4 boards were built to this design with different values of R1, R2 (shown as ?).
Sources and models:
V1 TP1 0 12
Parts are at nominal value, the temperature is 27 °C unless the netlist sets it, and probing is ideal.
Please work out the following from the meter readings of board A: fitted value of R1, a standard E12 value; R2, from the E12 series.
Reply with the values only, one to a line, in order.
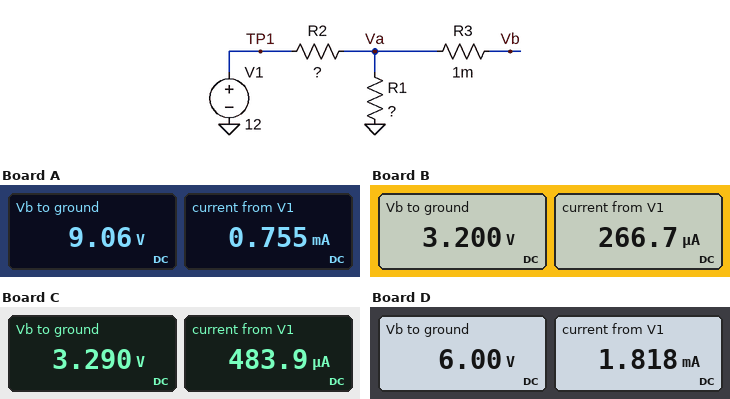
12 kΩ
3.9 kΩ
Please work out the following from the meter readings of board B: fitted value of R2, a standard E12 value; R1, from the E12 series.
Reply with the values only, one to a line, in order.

33 kΩ
12 kΩ
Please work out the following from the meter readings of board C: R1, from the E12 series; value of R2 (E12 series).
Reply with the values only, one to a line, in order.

6.8 kΩ
18 kΩ
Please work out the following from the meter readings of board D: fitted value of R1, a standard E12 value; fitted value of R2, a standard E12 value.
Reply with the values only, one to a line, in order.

3.3 kΩ
3.3 kΩ
